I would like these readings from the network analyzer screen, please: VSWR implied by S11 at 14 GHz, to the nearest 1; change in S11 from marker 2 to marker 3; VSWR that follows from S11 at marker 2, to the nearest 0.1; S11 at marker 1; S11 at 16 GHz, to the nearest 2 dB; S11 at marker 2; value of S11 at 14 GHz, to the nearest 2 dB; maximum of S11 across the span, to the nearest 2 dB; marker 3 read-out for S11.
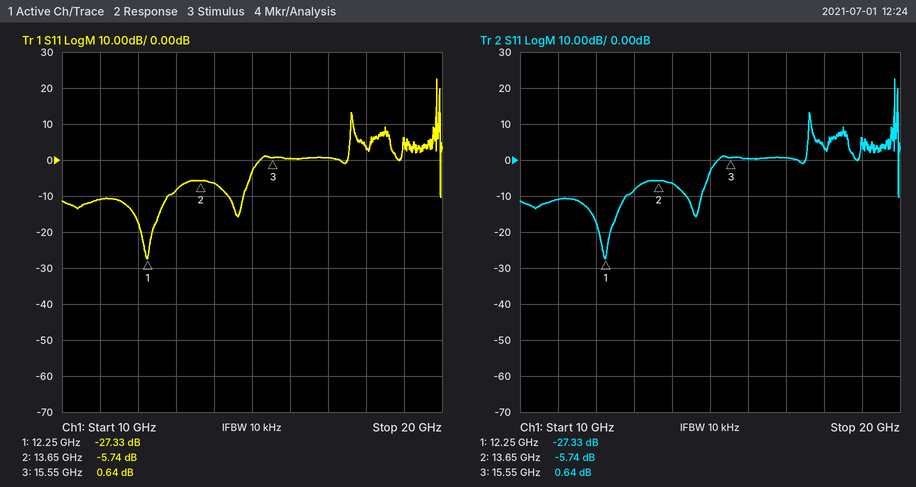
3
6.38 dB
3.1
-27.33 dB
0 dB
-5.74 dB
-6 dB
22 dB
0.64 dB
